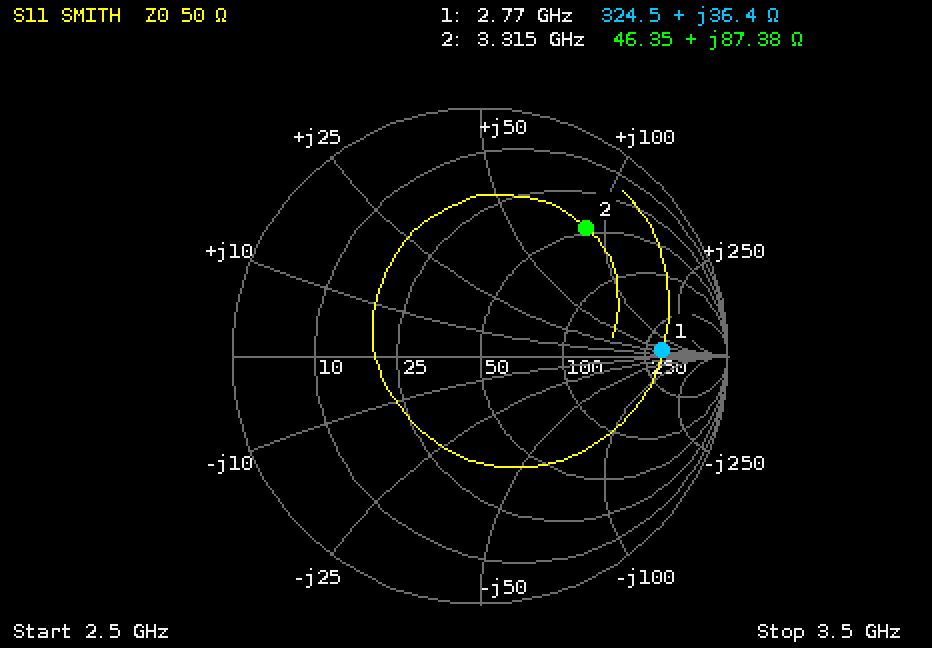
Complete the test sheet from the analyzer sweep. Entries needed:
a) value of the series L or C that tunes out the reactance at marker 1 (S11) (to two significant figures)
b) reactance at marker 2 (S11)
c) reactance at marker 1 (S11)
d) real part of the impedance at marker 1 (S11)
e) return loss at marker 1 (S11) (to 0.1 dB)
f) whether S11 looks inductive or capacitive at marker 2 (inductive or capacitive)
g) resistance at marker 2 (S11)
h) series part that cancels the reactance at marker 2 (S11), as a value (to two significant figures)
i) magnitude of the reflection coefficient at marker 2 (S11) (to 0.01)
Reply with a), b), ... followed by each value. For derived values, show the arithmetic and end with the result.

a) C = 1/(2π × 2.77 GHz × 36.4 Ω) ≈ 1.6 pF
b) +87.38 Ω
c) +36.4 Ω
d) 324.5 Ω
e) 2.7 dB
f) inductive
g) 46.35 Ω
h) C = 1/(2π × 3.315 GHz × 87.38 Ω) ≈ 549 fF, so 550 fF to two significant figures
i) 0.67
